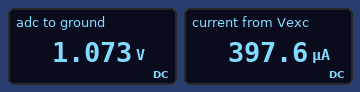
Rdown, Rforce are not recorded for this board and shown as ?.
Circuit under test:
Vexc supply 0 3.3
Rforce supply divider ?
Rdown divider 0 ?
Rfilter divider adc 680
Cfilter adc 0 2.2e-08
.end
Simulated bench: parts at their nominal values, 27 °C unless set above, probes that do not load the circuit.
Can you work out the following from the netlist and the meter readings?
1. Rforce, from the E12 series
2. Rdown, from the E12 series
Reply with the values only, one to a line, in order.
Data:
5.6 kΩ
2.7 kΩ
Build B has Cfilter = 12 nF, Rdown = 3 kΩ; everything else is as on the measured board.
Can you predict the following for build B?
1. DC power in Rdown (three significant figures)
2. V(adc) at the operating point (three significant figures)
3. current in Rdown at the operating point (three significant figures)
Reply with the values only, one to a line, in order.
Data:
442 µW
1.15 V
384 µA
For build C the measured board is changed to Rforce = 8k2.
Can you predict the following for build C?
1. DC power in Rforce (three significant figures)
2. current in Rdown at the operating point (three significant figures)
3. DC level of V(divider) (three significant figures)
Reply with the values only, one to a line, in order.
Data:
752 µW
303 µA
817 mV
